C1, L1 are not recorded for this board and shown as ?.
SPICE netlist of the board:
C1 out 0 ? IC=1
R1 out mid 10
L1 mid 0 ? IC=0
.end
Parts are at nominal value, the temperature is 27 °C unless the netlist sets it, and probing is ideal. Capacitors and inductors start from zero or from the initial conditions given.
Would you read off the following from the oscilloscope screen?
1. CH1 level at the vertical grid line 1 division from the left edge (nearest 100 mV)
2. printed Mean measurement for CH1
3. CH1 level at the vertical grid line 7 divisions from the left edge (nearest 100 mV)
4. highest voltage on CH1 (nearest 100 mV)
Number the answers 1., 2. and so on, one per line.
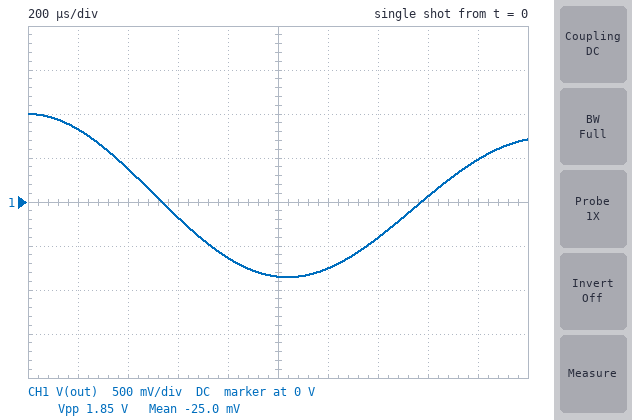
1. 800 mV
2. -25.0 mV
3. -400 mV
4. 1.0 V
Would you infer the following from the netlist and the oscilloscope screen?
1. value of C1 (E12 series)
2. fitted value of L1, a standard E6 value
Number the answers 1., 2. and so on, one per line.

1. 3.3 µF
2. 33 mH
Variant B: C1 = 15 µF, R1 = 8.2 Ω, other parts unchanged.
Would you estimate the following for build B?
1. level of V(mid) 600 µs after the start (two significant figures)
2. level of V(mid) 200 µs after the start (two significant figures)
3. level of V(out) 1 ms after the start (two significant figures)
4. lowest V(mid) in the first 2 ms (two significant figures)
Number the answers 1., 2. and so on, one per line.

1. 550 mV
2. 910 mV
3. 210 mV
4. -760 mV
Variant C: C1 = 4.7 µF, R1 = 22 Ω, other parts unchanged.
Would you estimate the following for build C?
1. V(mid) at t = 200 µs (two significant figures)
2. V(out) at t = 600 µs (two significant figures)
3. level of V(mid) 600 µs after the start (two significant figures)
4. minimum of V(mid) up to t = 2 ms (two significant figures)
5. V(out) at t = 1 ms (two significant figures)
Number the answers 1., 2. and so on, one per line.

1. 760 mV
2. 160 mV
3. -59 mV
4. -680 mV
5. -530 mV
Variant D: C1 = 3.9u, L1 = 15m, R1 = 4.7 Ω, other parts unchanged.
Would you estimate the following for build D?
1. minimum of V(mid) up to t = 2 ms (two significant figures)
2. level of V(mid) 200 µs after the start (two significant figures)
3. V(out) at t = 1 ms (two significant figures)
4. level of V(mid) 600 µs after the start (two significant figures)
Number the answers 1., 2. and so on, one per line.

1. -890 mV
2. 630 mV
3. -500 mV
4. -740 mV
